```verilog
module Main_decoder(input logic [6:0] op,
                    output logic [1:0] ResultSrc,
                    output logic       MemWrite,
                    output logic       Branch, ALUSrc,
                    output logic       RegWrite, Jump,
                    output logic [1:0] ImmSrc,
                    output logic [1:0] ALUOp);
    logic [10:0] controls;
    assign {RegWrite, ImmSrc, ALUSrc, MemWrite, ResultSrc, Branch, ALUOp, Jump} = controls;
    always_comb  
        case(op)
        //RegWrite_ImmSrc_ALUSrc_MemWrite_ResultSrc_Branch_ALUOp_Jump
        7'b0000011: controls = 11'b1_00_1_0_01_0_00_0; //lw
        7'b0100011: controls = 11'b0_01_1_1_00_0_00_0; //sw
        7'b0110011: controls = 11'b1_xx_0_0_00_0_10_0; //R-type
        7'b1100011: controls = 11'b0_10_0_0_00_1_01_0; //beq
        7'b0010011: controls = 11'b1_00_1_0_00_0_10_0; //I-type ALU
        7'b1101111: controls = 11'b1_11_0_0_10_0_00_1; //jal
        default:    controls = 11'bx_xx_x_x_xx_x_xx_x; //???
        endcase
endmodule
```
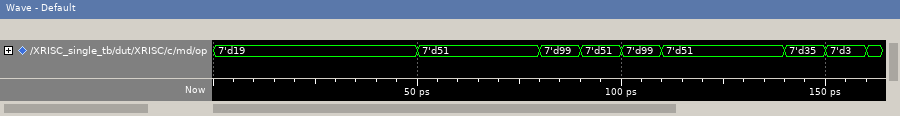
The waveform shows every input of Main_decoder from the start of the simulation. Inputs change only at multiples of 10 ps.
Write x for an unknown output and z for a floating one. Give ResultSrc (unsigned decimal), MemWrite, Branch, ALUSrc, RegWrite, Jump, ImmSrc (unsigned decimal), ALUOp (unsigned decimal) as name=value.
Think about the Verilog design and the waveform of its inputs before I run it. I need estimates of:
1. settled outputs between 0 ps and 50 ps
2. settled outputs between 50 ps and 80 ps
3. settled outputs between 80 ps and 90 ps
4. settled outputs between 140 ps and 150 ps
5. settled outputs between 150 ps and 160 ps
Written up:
ResultSrc=0, MemWrite=0, Branch=0, ALUSrc=1, RegWrite=1, Jump=0, ImmSrc=0, ALUOp=2
ResultSrc=0, MemWrite=0, Branch=0, ALUSrc=0, RegWrite=1, Jump=0, ImmSrc=x, ALUOp=2
ResultSrc=0, MemWrite=0, Branch=1, ALUSrc=0, RegWrite=0, Jump=0, ImmSrc=2, ALUOp=1
ResultSrc=0, MemWrite=1, Branch=0, ALUSrc=1, RegWrite=0, Jump=0, ImmSrc=1, ALUOp=0
ResultSrc=1, MemWrite=0, Branch=0, ALUSrc=1, RegWrite=1, Jump=0, ImmSrc=0, ALUOp=0
